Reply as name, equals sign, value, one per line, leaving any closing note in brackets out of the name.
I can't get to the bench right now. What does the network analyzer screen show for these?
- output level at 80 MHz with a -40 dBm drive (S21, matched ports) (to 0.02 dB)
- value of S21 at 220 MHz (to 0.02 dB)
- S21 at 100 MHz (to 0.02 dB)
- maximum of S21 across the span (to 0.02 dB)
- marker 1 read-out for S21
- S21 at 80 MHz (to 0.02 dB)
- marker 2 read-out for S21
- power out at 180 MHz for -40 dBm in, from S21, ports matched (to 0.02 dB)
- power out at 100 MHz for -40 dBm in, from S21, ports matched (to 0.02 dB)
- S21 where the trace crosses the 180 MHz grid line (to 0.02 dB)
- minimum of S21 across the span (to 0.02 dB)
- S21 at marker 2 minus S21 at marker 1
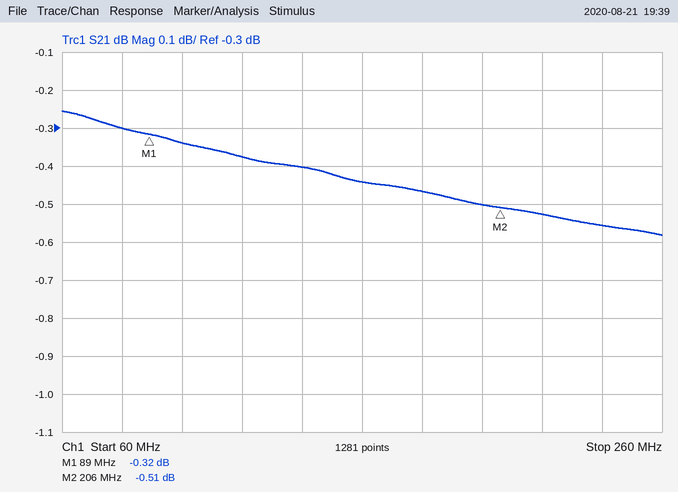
output level at 80 MHz with a -40 dBm drive (S21, matched ports) = -40.30 dBm
value of S21 at 220 MHz = -0.52 dB
S21 at 100 MHz = -0.34 dB
maximum of S21 across the span = -0.26 dB
marker 1 read-out for S21 = -0.32 dB
S21 at 80 MHz = -0.30 dB
marker 2 read-out for S21 = -0.51 dB
power out at 180 MHz for -40 dBm in, from S21, ports matched = -40.46 dBm
power out at 100 MHz for -40 dBm in, from S21, ports matched = -40.34 dBm
S21 where the trace crosses the 180 MHz grid line = -0.46 dB
minimum of S21 across the span = -0.58 dB
S21 at marker 2 minus S21 at marker 1 = -0.19 dB
